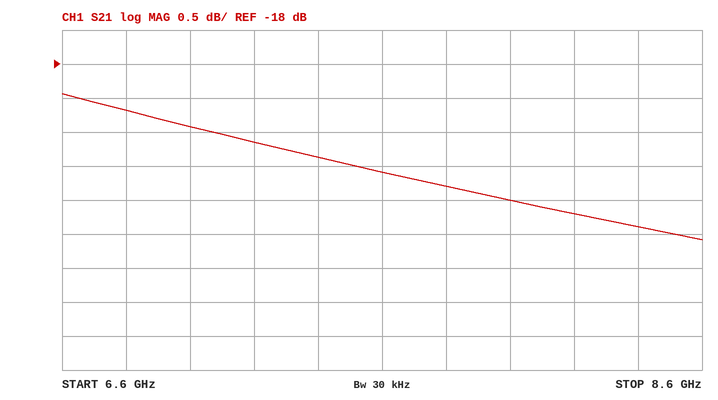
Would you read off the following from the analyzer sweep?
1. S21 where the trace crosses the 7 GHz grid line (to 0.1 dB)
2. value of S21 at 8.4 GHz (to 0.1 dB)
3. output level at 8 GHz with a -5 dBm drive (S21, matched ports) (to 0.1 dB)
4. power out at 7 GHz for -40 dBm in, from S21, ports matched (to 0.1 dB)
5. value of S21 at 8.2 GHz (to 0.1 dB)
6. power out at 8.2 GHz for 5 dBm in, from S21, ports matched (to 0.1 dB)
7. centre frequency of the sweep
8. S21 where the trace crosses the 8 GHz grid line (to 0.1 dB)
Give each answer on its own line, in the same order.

-18.9 dB
-20.4 dB
-25.0 dBm
-58.9 dBm
-20.2 dB
-15.2 dBm
7.6 GHz
-20.0 dB
